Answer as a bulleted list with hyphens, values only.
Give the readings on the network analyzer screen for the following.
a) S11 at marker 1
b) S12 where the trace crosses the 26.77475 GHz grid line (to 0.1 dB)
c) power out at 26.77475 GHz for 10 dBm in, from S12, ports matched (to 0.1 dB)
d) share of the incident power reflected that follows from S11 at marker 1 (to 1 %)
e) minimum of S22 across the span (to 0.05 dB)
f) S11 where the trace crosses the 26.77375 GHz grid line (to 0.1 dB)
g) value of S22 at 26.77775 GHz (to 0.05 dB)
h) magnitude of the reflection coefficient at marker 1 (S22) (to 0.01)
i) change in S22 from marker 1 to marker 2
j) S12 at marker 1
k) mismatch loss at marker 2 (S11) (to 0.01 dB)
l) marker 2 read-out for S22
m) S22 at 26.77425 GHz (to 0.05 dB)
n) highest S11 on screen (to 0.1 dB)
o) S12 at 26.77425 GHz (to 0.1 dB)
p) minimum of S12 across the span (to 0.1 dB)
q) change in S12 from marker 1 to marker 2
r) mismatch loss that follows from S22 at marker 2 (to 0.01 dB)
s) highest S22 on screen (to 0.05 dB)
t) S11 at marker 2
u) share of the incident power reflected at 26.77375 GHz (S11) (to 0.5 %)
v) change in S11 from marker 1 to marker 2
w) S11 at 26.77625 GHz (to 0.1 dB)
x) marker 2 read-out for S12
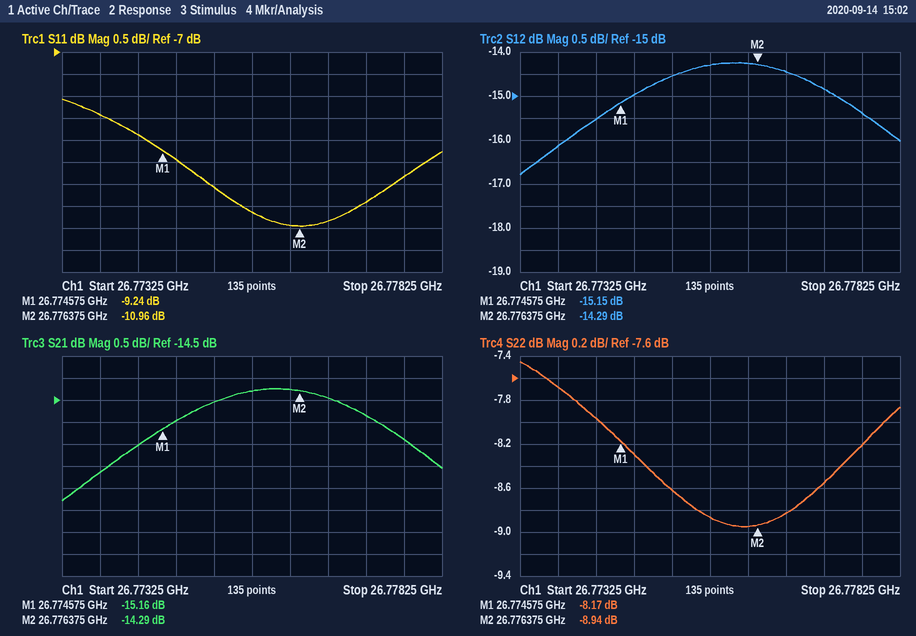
- -9.24 dB
- -15.0 dB
- -5.0 dBm
- 12 %
- -8.95 dB
- -8.4 dB
- -8.20 dB
- 0.39
- -0.77 dB
- -15.15 dB
- 0.36 dB
- -8.94 dB
- -7.95 dB
- -8.1 dB
- -15.5 dB
- -16.8 dB
- 0.86 dB
- 0.59 dB
- -7.45 dB
- -10.96 dB
- 14.5 %
- -1.72 dB
- -10.9 dB
- -14.29 dB
